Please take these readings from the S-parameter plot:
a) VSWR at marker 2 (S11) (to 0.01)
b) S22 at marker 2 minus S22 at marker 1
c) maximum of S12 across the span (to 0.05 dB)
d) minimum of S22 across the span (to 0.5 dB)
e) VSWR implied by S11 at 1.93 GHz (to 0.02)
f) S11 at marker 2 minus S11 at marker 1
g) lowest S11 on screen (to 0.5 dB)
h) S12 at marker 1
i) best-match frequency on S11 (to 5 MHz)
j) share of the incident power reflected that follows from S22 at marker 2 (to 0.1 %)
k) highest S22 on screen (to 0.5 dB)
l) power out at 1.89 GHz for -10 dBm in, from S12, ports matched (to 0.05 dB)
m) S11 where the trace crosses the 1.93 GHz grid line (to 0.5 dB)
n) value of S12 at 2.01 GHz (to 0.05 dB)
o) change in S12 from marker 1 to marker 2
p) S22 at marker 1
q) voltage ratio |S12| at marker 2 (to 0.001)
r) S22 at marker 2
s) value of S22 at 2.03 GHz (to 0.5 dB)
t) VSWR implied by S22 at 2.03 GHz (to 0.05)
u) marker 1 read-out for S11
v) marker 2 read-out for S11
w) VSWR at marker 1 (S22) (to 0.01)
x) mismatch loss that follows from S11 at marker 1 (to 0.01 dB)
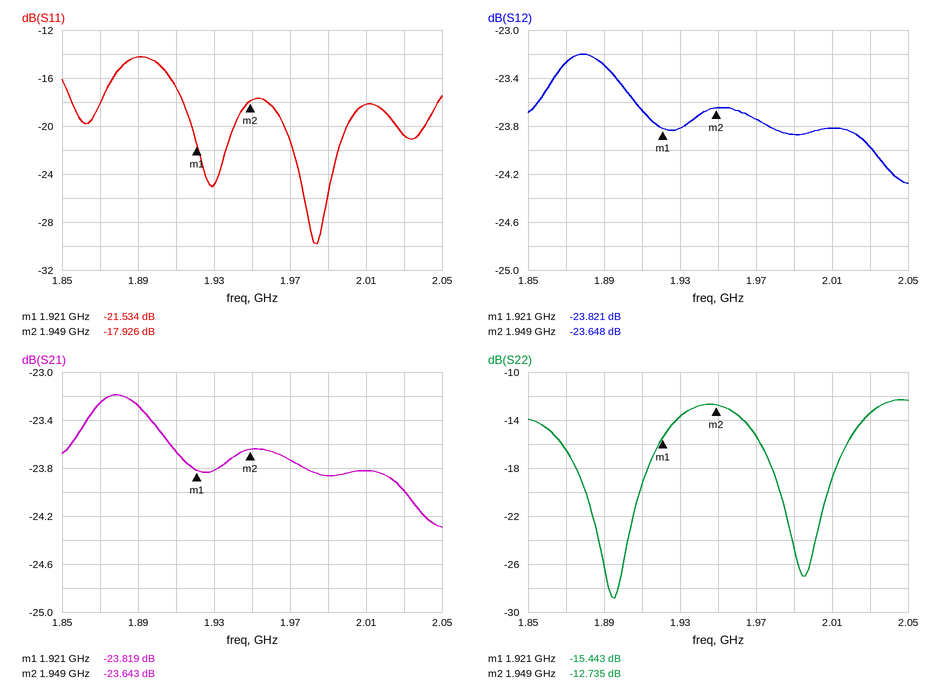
1.29
2.708 dB
-23.20 dB
-29.0 dB
1.12
3.608 dB
-30.0 dB
-23.821 dB
1.985 GHz
5.3 %
-12.5 dB
-33.30 dBm
-25.0 dB
-23.80 dB
0.173 dB
-15.443 dB
0.066
-12.735 dB
-13.5 dB
1.55
-21.534 dB
-17.926 dB
1.41
0.03 dB
